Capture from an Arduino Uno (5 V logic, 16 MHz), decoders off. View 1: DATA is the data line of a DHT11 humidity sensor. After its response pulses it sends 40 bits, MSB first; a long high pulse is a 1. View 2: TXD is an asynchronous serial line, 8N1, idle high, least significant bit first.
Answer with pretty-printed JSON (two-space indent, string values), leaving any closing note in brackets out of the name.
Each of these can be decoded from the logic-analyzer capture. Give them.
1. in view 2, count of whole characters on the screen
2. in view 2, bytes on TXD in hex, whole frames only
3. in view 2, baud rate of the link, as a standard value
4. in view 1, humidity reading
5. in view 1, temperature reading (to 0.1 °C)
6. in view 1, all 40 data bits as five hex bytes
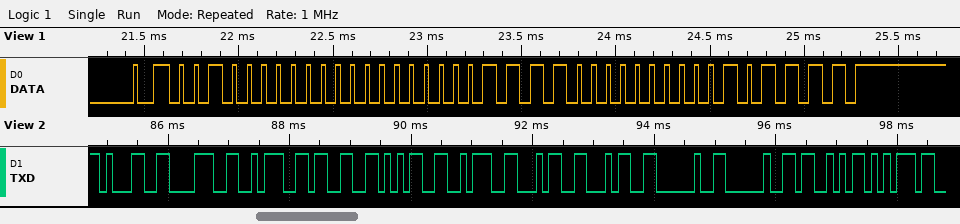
{
  "in view 2, count of whole characters on the screen": "12",
  "in view 2, bytes on TXD in hex, whole frames only": "0x31 0x38 0x3A 0x33 0x35 0x3A 0x34 0x34 0x20 0x20 0x53 0x75",
  "in view 2, baud rate of the link, as a standard value": "9600 baud",
  "in view 1, humidity reading": "32 %",
  "in view 1, temperature reading": "15.0 °C",
  "in view 1, all 40 data bits as five hex bytes": "20 00 0F 00 2F"
}
